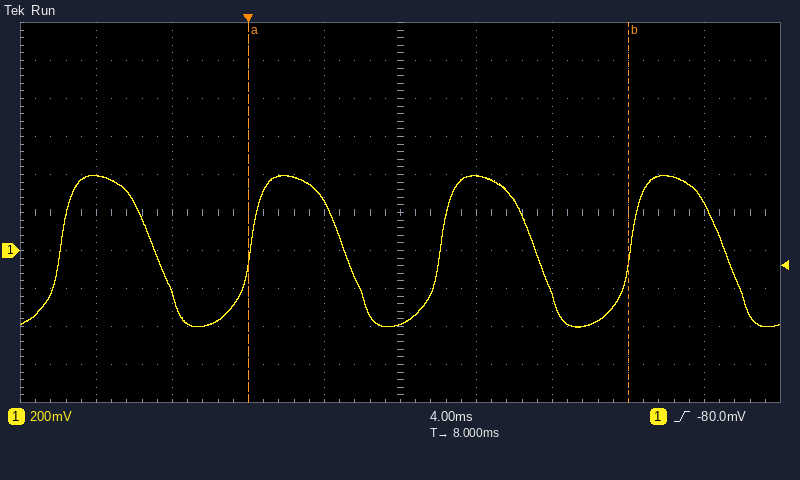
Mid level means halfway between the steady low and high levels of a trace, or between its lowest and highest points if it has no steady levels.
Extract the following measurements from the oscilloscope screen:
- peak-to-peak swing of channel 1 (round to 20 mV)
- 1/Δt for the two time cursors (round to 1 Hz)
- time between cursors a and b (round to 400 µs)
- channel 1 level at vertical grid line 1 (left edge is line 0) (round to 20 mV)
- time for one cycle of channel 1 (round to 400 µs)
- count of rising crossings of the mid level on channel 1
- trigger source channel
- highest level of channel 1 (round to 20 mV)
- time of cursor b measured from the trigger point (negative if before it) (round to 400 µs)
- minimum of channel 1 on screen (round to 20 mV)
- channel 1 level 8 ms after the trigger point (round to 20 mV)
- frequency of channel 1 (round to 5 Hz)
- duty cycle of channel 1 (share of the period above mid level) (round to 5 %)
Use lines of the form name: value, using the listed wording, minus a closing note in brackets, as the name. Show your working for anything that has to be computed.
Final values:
peak-to-peak swing of channel 1: 400 mV − (-400 mV) = 800 mV
1/Δt for the two time cursors: 1 / 20.0 ms ≈ 50 Hz
time between cursors a and b: 20.0 ms
channel 1 level at vertical grid line 1 (left edge is line 0): 400 mV
time for one cycle of channel 1: 10.0 ms
count of rising crossings of the mid level on channel 1: 4
trigger source channel: channel 1
highest level of channel 1: 400 mV
time of cursor b measured from the trigger point (negative if before it): +20.0 ms
minimum of channel 1 on screen: -400 mV
channel 1 level 8 ms after the trigger point: -380 mV
frequency of channel 1: 1 / 10.0 ms ≈ 100 Hz
duty cycle of channel 1 (share of the period above mid level): 50 %
